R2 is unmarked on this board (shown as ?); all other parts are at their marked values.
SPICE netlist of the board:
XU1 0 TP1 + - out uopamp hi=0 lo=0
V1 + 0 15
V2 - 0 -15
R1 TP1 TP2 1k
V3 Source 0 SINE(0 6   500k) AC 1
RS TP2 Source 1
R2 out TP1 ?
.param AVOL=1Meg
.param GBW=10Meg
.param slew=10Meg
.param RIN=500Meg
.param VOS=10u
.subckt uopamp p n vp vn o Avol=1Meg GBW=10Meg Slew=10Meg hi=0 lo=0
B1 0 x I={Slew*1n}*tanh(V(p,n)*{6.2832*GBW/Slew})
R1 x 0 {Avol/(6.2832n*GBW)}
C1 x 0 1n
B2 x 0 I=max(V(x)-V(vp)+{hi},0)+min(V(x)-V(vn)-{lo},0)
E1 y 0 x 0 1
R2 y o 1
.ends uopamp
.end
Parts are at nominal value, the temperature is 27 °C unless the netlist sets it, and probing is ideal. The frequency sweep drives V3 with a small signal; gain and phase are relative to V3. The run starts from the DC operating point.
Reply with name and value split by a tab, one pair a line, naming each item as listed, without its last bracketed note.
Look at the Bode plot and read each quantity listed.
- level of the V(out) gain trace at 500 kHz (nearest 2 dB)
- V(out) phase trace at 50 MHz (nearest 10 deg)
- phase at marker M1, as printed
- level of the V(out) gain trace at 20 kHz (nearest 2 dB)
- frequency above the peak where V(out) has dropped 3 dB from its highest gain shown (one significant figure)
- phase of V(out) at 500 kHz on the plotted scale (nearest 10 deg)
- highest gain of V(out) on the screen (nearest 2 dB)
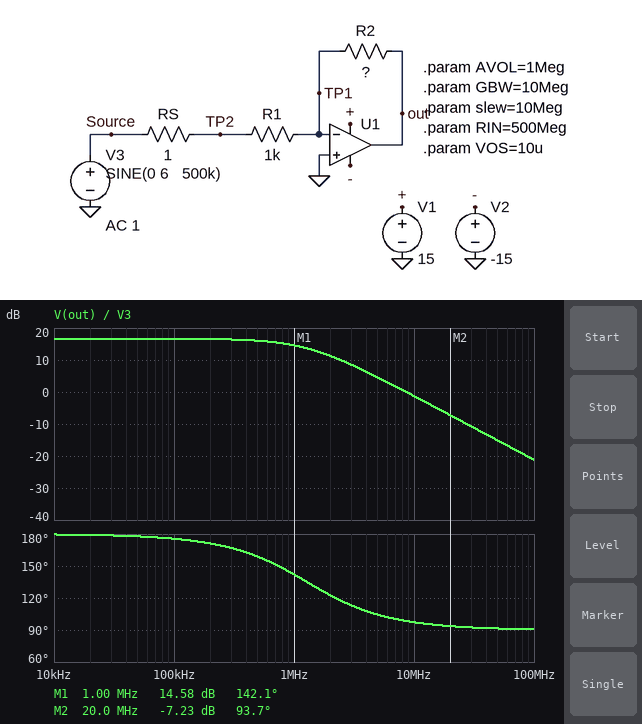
level of the V(out) gain trace at 500 kHz	16 dB
V(out) phase trace at 50 MHz	90 deg
phase at marker M1, as printed	142.1 deg
level of the V(out) gain trace at 20 kHz	16 dB
frequency above the peak where V(out) has dropped 3 dB from its highest gain shown	1 MHz
phase of V(out) at 500 kHz on the plotted scale	160 deg
highest gain of V(out) on the screen	16 dB
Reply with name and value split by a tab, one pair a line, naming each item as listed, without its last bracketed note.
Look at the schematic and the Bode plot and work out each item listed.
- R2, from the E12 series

R2, from the E12 series	6.8 kΩ
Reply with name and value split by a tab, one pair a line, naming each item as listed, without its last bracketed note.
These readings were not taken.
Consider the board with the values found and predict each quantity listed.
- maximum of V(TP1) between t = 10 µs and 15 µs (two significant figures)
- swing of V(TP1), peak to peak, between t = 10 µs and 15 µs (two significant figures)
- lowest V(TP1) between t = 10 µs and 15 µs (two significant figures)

maximum of V(TP1) between t = 10 µs and 15 µs	5.1 V
swing of V(TP1), peak to peak, between t = 10 µs and 15 µs	10 V
lowest V(TP1) between t = 10 µs and 15 µs	-5.3 V
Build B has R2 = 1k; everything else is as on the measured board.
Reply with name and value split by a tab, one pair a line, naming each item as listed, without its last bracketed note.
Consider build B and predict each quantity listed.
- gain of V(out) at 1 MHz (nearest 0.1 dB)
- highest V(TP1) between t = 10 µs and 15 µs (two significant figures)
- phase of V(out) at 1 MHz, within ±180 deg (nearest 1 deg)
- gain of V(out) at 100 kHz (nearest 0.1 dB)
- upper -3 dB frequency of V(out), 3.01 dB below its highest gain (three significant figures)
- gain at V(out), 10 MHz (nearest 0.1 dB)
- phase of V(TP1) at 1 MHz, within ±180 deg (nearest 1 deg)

gain of V(out) at 1 MHz	-0.2 dB
highest V(TP1) between t = 10 µs and 15 µs	2.0 V
phase of V(out) at 1 MHz, within ±180 deg	169 deg
gain of V(out) at 100 kHz	0 dB
upper -3 dB frequency of V(out), 3.01 dB below its highest gain	5.00 MHz
gain at V(out), 10 MHz	-7.0 dB
phase of V(TP1) at 1 MHz, within ±180 deg	79 deg
